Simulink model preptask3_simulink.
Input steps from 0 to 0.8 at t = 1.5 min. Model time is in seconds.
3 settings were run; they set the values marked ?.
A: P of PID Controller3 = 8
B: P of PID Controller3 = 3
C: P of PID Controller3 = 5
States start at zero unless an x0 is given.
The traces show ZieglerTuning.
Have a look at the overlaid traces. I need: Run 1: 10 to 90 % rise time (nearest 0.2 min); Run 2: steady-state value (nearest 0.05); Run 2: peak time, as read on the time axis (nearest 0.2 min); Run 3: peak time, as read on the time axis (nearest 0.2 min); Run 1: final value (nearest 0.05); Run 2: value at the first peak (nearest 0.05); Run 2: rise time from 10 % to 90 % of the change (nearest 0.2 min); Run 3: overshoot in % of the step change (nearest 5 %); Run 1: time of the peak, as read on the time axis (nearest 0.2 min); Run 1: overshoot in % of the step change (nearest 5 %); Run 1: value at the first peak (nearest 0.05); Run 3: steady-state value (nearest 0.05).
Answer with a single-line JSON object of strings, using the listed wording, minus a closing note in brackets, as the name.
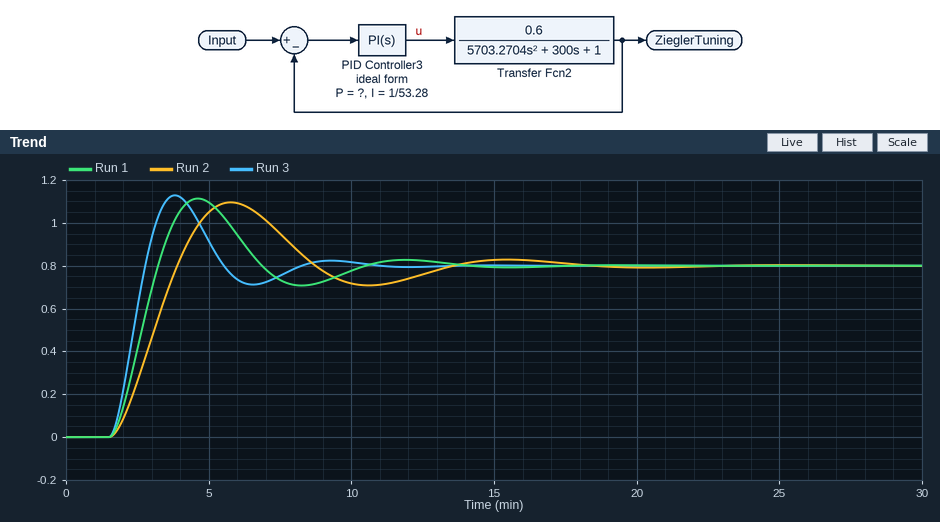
{"Run 1: 10 to 90 % rise time": "1.2 min", "Run 2: steady-state value": "0.80", "Run 2: peak time, as read on the time axis": "5.8 min", "Run 3: peak time, as read on the time axis": "3.8 min", "Run 1: final value": "0.80", "Run 2: value at the first peak": "1.10", "Run 2: rise time from 10 % to 90 % of the change": "1.6 min", "Run 3: overshoot in % of the step change": "40 %", "Run 1: time of the peak, as read on the time axis": "4.6 min", "Run 1: overshoot in % of the step change": "40 %", "Run 1: value at the first peak": "1.10", "Run 3: steady-state value": "0.80"}
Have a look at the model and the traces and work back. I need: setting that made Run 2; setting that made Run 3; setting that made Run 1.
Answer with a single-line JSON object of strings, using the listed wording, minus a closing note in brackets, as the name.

{"setting that made Run 2": "B", "setting that made Run 3": "A", "setting that made Run 1": "C"}
